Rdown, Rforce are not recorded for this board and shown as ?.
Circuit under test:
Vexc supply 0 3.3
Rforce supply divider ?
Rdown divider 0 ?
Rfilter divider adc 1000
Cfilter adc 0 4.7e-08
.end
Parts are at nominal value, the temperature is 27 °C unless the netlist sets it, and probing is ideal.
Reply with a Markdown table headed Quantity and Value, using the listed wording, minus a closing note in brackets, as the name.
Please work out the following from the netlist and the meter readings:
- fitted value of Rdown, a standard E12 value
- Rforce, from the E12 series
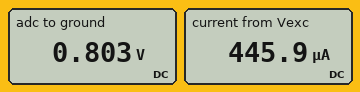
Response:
| Quantity | Value |
|---|---|
| fitted value of Rdown, a standard E12 value | 1.8 kΩ |
| Rforce, from the E12 series | 5.6 kΩ |
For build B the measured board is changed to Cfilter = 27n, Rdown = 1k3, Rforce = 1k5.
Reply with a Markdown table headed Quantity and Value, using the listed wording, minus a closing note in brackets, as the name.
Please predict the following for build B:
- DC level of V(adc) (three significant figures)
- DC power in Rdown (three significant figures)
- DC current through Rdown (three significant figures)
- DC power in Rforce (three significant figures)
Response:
| Quantity | Value |
|---|---|
| DC level of V(adc) | 1.53 V |
| DC power in Rdown | 1.81 mW |
| DC current through Rdown | 1.18 mA |
| DC power in Rforce | 2.08 mW |
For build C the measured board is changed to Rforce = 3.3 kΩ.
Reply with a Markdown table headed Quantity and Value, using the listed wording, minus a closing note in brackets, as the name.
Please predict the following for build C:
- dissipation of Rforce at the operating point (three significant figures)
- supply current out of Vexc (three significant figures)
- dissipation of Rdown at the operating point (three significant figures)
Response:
| Quantity | Value |
|---|---|
| dissipation of Rforce at the operating point | 1.38 mW |
| supply current out of Vexc | 647 µA |
| dissipation of Rdown at the operating point | 754 µW |
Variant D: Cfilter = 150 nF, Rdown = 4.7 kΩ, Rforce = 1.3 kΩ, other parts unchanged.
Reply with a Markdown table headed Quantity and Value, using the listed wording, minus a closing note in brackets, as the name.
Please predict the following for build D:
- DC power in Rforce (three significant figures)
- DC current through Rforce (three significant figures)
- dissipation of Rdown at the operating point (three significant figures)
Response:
| Quantity | Value |
|---|---|
| DC power in Rforce | 393 µW |
| DC current through Rforce | 550 µA |
| dissipation of Rdown at the operating point | 1.42 mW |
